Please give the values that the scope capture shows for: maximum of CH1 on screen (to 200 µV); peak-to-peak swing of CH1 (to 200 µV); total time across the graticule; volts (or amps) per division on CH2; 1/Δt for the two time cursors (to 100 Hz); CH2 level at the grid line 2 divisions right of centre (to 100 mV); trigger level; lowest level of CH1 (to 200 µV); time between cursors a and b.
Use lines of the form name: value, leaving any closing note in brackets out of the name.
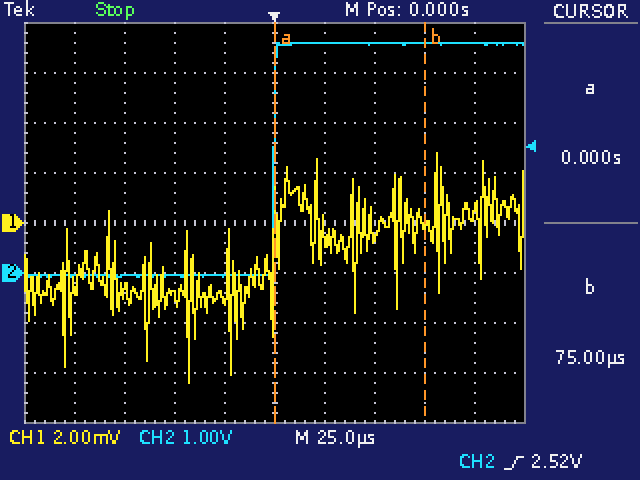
maximum of CH1 on screen: 2.8 mV
peak-to-peak swing of CH1: 9.2 mV
total time across the graticule: 250 µs
volts (or amps) per division on CH2: 1 V
1/Δt for the two time cursors: 13.3 kHz
CH2 level at the grid line 2 divisions right of centre: 4.6 V
trigger level: 2.52 V
lowest level of CH1: -6.4 mV
time between cursors a and b: 75.0 µs
